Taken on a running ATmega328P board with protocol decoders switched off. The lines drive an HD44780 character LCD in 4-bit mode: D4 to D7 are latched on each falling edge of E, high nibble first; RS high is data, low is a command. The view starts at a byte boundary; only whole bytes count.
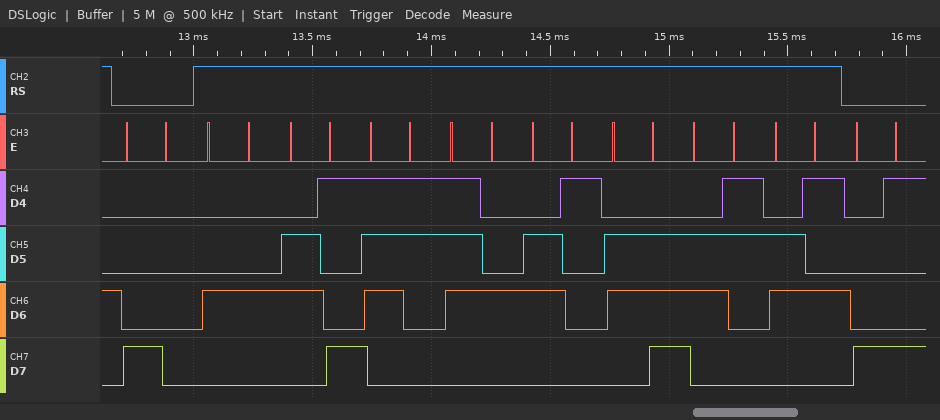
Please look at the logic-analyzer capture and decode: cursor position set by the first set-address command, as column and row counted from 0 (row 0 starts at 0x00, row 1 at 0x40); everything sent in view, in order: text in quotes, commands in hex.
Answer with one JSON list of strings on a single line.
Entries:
["column 0, row 0", "0x80 \"Distance\" 0x89"]
